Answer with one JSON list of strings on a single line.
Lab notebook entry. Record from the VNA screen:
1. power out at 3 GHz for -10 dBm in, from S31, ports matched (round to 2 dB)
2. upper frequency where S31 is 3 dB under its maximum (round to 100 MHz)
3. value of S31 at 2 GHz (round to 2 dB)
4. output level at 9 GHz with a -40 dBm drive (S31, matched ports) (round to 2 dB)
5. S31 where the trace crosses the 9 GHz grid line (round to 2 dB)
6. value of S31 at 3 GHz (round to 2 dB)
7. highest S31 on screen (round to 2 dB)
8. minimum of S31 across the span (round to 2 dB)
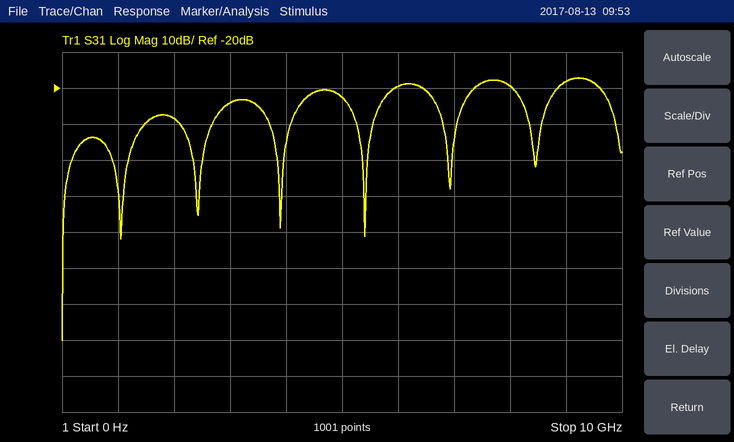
["-34 dBm", "9.6 GHz", "-28 dB", "-58 dBm", "-18 dB", "-24 dB", "-18 dB", "-90 dB"]
